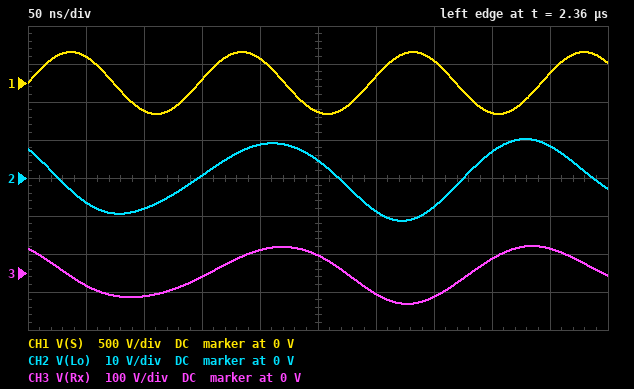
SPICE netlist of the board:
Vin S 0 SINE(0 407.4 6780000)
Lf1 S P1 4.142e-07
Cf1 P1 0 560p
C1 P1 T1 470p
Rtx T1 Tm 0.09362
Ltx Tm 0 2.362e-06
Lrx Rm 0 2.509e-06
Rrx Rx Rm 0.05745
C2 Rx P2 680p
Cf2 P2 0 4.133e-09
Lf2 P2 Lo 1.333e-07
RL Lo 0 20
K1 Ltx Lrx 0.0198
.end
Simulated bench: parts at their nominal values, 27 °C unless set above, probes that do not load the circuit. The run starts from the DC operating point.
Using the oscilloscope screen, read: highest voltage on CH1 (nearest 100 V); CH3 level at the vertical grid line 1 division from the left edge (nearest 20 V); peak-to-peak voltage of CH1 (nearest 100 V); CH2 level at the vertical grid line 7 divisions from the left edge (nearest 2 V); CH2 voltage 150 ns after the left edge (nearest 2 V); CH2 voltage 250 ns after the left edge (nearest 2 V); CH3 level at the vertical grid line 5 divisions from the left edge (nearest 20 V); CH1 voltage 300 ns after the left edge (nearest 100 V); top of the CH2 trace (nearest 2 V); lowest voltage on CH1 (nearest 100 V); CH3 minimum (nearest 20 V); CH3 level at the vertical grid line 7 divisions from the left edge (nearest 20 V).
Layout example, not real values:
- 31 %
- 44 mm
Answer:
- 400 V
- -40 V
- 800 V
- -8 V
- 0 V
- 4 V
- 40 V
- 100 V
- 10 V
- -400 V
- -80 V
- -60 V
